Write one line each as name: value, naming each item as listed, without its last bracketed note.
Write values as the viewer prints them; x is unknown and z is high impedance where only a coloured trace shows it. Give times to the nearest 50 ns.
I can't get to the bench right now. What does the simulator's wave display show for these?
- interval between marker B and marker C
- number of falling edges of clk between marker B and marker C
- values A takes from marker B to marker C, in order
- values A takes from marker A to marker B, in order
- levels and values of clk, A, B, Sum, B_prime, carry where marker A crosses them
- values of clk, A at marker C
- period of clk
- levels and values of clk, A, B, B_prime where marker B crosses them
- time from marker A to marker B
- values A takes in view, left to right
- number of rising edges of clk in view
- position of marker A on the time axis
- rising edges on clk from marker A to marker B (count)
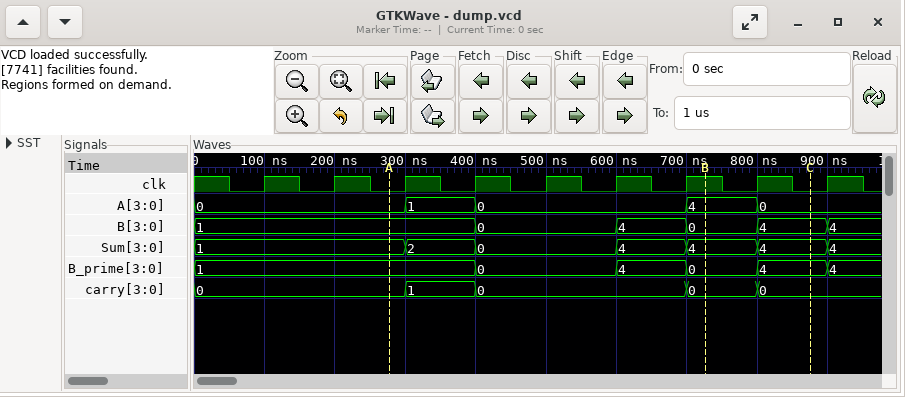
interval between marker B and marker C: 150 ns
number of falling edges of clk between marker B and marker C: 2
values A takes from marker B to marker C, in order: 4, 0
values A takes from marker A to marker B, in order: 0, 1, 0, 4
levels and values of clk, A, B, Sum, B_prime, carry where marker A crosses them: clk=0, A=0, B=1, Sum=1, B_prime=1, carry=0
values of clk, A at marker C: clk=0, A=0
period of clk: 100 ns
levels and values of clk, A, B, B_prime where marker B crosses them: clk=1, A=4, B=0, B_prime=0
time from marker A to marker B: 450 ns
values A takes in view, left to right: 0, 1, 0, 4, 0
number of rising edges of clk in view: 9
position of marker A on the time axis: 300 ns
rising edges on clk from marker A to marker B: 5
